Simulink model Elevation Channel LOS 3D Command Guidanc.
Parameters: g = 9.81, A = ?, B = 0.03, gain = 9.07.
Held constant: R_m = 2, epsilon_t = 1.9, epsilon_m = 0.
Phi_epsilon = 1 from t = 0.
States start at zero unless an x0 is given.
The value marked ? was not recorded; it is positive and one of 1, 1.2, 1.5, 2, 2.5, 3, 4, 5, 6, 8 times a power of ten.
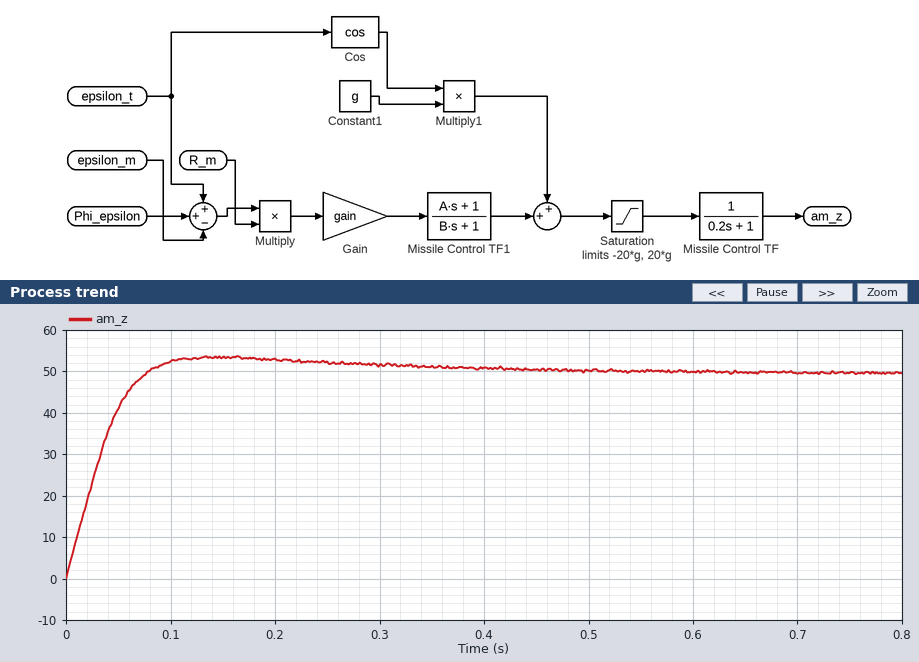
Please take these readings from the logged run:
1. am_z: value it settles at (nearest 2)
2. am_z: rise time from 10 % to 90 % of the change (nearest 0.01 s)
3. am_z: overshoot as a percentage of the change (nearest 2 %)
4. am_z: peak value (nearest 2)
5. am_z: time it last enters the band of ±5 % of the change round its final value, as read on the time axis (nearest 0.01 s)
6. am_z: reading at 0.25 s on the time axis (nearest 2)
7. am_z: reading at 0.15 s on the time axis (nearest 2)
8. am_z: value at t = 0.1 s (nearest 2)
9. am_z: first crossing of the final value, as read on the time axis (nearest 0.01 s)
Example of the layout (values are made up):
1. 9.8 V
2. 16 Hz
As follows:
1. 50
2. 0.05 s
3. 8 %
4. 54
5. 0.27 s
6. 52
7. 54
8. 52
9. 0.08 s
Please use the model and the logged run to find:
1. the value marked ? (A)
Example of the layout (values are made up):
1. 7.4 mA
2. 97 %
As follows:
1. 0.3
